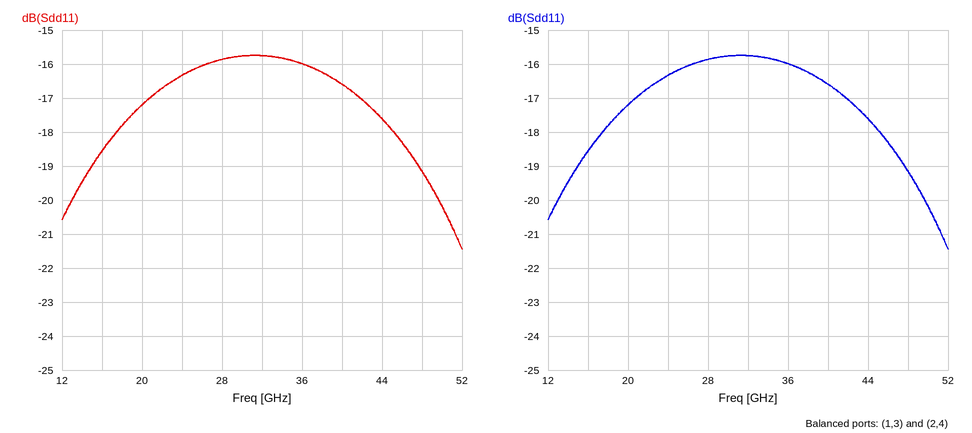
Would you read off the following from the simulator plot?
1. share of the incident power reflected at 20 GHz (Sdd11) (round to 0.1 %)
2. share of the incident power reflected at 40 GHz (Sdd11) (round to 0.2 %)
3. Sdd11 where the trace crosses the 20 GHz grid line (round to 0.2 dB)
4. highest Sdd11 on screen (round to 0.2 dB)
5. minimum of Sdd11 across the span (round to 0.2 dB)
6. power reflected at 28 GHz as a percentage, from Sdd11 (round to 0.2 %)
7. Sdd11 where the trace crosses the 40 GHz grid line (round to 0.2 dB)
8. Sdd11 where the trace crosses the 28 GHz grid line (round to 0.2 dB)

1.9 %
2.2 %
-17.2 dB
-15.8 dB
-21.4 dB
2.6 %
-16.6 dB
-15.8 dB
